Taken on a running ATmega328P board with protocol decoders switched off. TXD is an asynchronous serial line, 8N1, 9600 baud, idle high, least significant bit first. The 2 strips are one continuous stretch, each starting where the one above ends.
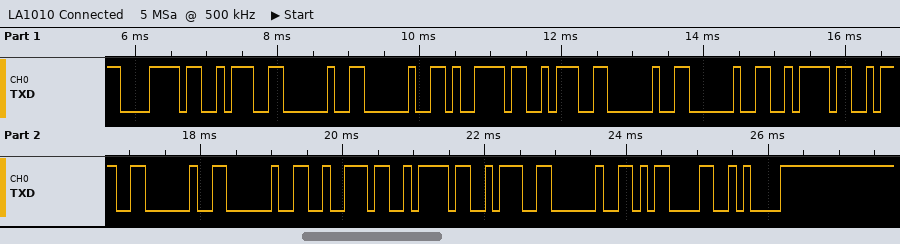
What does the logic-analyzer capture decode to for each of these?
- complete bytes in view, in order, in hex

78 3A 20 20 79 3A 20 20 7A 3A 20 20 72 7A 3A 20 0D 0A
